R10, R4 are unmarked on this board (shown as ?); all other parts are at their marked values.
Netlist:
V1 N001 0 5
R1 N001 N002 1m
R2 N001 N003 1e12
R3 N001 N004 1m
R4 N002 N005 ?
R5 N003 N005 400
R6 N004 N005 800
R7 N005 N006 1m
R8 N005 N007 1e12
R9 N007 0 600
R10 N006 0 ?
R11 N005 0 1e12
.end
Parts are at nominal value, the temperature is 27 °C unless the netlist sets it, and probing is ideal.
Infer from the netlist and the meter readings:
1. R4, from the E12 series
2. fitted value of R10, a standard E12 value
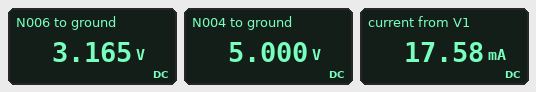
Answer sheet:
120 Ω
180 Ω
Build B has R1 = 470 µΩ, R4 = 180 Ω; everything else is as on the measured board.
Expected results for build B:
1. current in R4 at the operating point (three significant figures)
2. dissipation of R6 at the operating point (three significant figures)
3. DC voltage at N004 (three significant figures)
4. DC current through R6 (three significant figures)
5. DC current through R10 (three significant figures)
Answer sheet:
12.5 mA
6.31 mW
5.00 V
2.81 mA
15.3 mA
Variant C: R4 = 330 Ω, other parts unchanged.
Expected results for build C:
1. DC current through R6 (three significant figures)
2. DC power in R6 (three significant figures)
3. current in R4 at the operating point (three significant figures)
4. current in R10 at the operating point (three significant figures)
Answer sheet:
3.53 mA
9.97 mW
8.56 mA
12.1 mA
